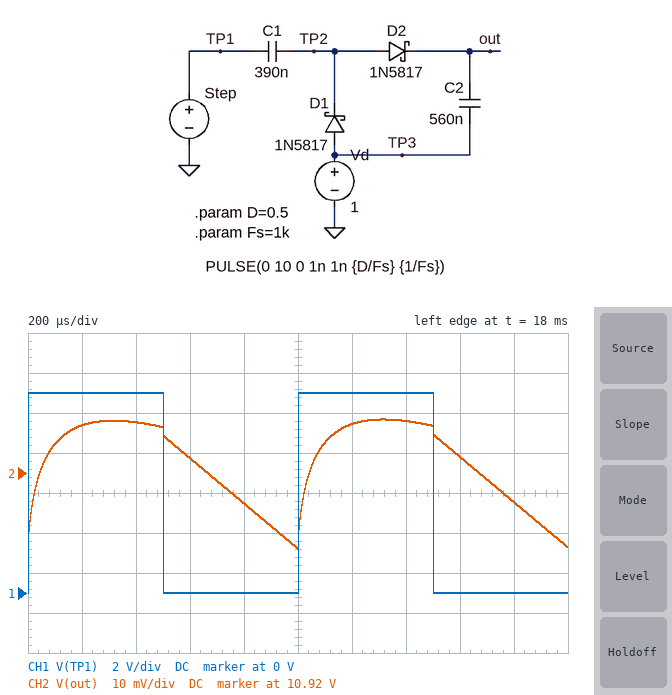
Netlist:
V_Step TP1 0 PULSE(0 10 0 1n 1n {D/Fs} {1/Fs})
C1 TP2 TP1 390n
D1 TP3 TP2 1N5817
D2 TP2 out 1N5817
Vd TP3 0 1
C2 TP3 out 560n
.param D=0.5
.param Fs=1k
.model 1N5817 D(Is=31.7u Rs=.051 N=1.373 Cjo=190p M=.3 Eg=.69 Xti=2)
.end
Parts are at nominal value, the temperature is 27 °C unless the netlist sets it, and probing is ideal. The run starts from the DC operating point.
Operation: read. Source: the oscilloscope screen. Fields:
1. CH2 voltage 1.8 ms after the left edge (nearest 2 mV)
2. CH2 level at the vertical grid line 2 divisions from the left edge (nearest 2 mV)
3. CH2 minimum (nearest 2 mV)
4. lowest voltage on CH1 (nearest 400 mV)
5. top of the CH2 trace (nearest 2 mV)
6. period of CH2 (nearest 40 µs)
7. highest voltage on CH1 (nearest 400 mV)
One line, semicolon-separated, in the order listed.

10.912 V; 10.932 V; 10.900 V; 0 V; 10.934 V; 1.00 ms; 10.0 V
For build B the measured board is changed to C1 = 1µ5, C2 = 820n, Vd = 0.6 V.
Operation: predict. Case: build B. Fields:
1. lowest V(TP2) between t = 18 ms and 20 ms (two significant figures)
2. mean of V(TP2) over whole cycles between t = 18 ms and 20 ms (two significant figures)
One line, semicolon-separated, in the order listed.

560 mV; 5.6 V
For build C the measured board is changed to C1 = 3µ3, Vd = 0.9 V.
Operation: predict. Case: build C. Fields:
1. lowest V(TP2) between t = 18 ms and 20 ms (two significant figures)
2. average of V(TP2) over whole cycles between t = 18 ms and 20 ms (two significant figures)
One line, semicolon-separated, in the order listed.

870 mV; 5.9 V
